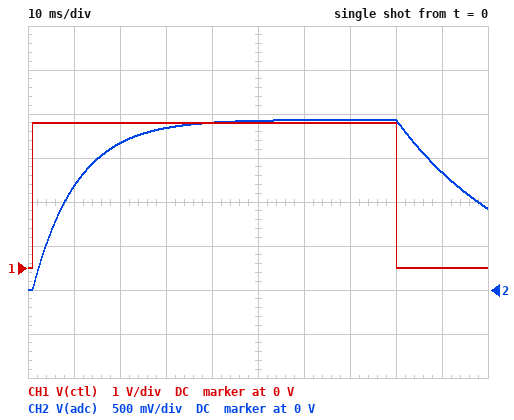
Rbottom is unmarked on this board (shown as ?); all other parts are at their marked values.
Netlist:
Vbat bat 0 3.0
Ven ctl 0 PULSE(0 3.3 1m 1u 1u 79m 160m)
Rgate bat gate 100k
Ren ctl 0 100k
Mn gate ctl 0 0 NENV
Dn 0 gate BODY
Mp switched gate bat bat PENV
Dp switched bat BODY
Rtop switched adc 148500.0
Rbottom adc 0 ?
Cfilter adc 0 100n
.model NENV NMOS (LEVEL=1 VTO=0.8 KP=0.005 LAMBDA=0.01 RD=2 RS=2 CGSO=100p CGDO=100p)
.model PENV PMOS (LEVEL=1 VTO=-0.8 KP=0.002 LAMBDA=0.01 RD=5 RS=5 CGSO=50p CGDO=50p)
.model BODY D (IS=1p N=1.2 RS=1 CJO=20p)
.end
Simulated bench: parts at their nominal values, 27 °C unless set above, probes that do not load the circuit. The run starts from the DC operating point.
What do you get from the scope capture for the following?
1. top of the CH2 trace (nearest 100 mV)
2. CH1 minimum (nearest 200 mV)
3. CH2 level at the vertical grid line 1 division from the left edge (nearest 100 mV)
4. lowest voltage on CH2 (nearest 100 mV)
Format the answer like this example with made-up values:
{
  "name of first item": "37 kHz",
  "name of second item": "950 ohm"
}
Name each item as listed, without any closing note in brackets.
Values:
{
  "top of the CH2 trace": "1.9 V",
  "CH1 minimum": "0 V",
  "CH2 level at the vertical grid line 1 division from the left edge": "1.2 V",
  "lowest voltage on CH2": "0 V"
}
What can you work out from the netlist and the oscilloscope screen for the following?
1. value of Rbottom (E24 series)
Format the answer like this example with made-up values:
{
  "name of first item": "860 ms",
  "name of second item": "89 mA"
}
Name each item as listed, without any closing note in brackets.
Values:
{
  "value of Rbottom": "270 kΩ"
}
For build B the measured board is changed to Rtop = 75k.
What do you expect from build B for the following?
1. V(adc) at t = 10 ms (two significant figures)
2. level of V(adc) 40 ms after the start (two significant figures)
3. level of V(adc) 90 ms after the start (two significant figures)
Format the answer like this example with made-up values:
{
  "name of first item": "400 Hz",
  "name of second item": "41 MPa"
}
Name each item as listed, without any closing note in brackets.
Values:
{
  "V(adc) at t = 10 ms": "1.8 V",
  "level of V(adc) 40 ms after the start": "2.3 V",
  "level of V(adc) 90 ms after the start": "1.6 V"
}
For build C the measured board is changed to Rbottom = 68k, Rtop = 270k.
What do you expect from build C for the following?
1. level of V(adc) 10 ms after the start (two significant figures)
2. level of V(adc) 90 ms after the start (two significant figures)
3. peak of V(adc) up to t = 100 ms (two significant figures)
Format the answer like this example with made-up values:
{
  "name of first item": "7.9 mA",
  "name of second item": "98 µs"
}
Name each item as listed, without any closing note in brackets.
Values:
{
  "level of V(adc) 10 ms after the start": "490 mV",
  "level of V(adc) 90 ms after the start": "140 mV",
  "peak of V(adc) up to t = 100 ms": "600 mV"
}
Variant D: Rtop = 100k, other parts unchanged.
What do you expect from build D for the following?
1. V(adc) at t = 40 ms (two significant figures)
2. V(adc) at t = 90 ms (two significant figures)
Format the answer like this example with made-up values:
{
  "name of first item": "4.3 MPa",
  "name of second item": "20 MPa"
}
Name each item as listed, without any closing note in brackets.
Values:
{
  "V(adc) at t = 40 ms": "2.2 V",
  "V(adc) at t = 90 ms": "1.5 V"
}
